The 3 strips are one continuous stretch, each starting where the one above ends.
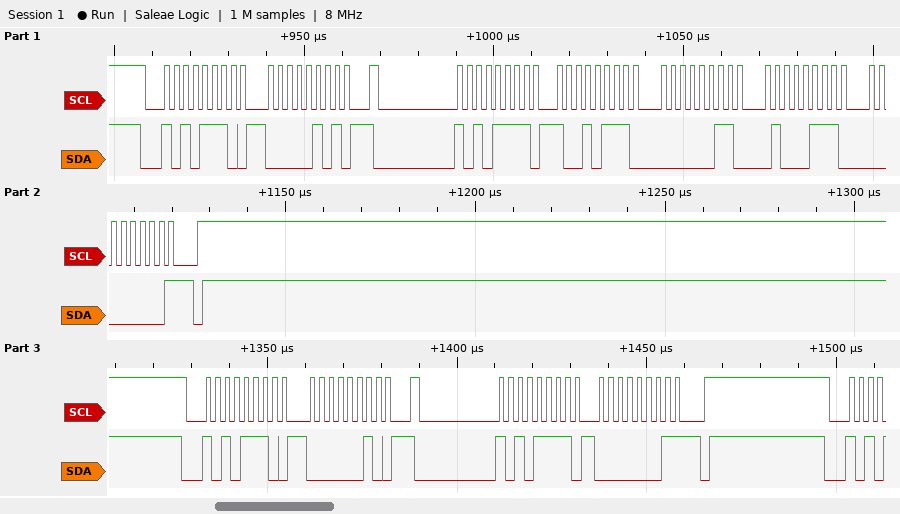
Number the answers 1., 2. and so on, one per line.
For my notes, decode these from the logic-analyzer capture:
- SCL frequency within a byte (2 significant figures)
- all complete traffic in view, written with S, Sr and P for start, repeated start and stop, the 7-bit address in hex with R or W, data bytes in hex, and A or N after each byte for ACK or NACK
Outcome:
1. 400 kHz
2. S 57W A 05 A Sr 57R A 97 A 03 A 47 A 00 N P S 57W A 02 A Sr 57R A 01 N P
